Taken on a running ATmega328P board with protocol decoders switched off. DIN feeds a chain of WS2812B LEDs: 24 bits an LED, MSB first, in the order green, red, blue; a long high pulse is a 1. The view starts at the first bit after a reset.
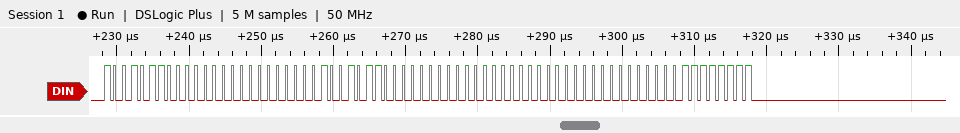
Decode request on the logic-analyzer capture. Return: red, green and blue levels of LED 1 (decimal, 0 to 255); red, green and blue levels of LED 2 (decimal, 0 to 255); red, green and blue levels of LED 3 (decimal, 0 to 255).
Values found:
0, 150, 0
0, 150, 0
0, 0, 255
